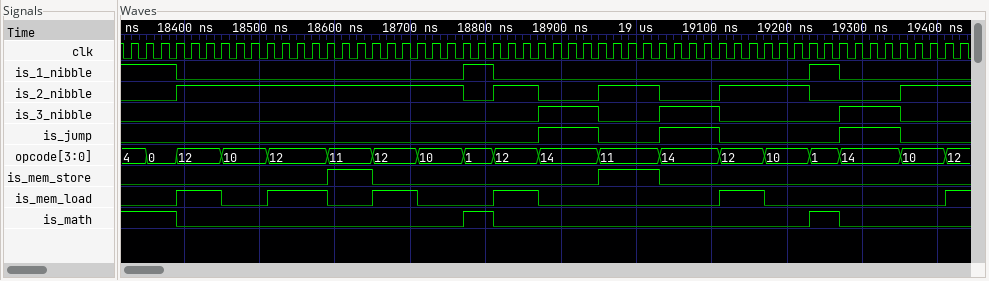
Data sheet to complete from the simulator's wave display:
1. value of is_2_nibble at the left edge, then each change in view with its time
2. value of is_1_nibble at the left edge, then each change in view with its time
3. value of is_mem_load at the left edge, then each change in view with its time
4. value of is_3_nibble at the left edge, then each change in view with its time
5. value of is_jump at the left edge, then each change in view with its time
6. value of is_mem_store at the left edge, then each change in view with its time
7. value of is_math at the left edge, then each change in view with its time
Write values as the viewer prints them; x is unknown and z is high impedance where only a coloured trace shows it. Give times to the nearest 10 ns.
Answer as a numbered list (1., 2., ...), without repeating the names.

1. 0, 1 at 18390 ns, 0 at 18770 ns, 1 at 18810 ns, 0 at 18870 ns, 1 at 18950 ns, 0 at 19030 ns, 1 at 19110 ns, 0 at 19230 ns, 1 at 19350 ns
2. 1, 0 at 18390 ns, 1 at 18770 ns, 0 at 18810 ns, 1 at 19230 ns, 0 at 19270 ns
3. 0, 1 at 18390 ns, 0 at 18450 ns, 1 at 18510 ns, 0 at 18590 ns, 1 at 18650 ns, 0 at 18710 ns, 1 at 18810 ns, 0 at 18870 ns, 1 at 19110 ns, 0 at 19170 ns, 1 at 19410 ns
4. 0, 1 at 18870 ns, 0 at 18950 ns, 1 at 19030 ns, 0 at 19110 ns, 1 at 19270 ns, 0 at 19350 ns
5. 0, 1 at 18870 ns, 0 at 18950 ns, 1 at 19030 ns, 0 at 19110 ns, 1 at 19270 ns, 0 at 19350 ns
6. 0, 1 at 18590 ns, 0 at 18650 ns, 1 at 18950 ns, 0 at 19030 ns
7. 1, 0 at 18390 ns, 1 at 18770 ns, 0 at 18810 ns, 1 at 19230 ns, 0 at 19270 ns
